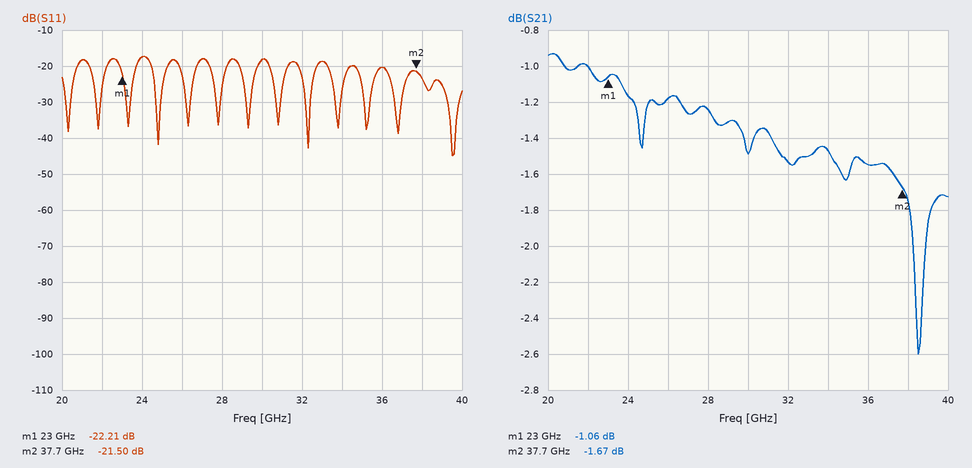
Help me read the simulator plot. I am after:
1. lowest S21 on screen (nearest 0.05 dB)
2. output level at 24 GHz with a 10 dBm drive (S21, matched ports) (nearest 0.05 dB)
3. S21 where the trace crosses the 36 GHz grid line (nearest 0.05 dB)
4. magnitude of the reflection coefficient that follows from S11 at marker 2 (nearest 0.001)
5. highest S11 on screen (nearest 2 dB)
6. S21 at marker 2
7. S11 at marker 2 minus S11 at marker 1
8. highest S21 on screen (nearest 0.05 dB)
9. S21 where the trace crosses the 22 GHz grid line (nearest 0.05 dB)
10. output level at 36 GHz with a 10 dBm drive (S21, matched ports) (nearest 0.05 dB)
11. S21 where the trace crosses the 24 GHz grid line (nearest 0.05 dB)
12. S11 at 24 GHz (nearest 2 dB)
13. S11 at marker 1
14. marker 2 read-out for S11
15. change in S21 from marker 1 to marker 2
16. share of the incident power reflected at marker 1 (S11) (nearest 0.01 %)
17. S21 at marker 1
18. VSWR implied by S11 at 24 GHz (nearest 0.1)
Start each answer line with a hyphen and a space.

- -2.60 dB
- 8.85 dBm
- -1.55 dB
- 0.084
- -18 dB
- -1.67 dB
- 0.71 dB
- -0.95 dB
- -1.00 dB
- 8.45 dBm
- -1.15 dB
- -18 dB
- -22.21 dB
- -21.50 dB
- -0.61 dB
- 0.60 %
- -1.06 dB
- 1.3
